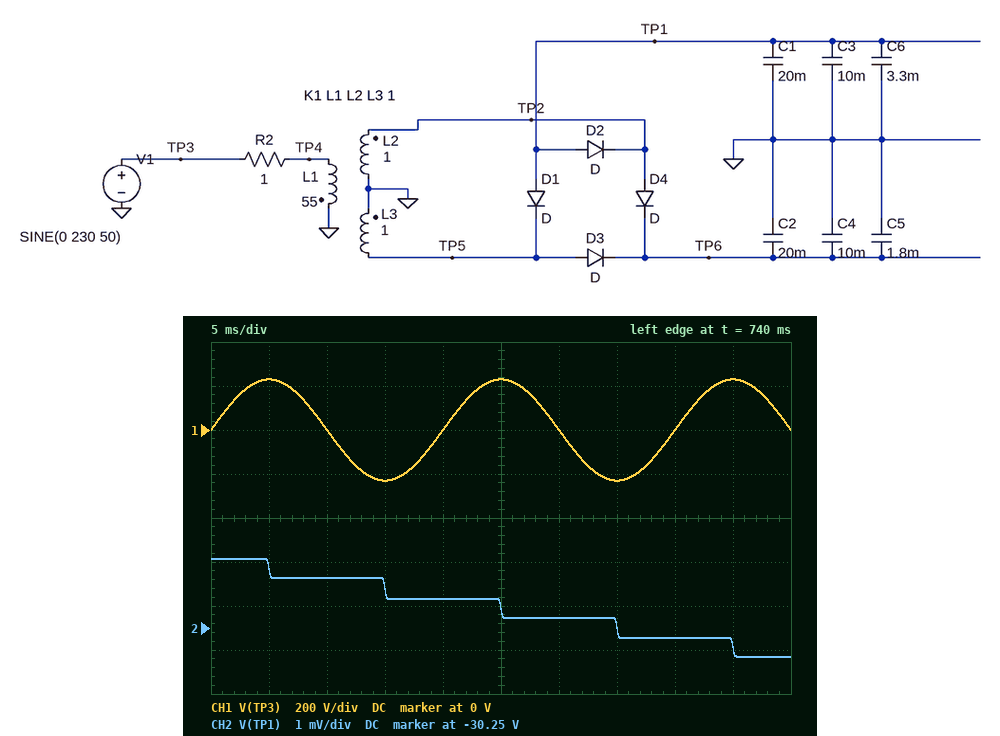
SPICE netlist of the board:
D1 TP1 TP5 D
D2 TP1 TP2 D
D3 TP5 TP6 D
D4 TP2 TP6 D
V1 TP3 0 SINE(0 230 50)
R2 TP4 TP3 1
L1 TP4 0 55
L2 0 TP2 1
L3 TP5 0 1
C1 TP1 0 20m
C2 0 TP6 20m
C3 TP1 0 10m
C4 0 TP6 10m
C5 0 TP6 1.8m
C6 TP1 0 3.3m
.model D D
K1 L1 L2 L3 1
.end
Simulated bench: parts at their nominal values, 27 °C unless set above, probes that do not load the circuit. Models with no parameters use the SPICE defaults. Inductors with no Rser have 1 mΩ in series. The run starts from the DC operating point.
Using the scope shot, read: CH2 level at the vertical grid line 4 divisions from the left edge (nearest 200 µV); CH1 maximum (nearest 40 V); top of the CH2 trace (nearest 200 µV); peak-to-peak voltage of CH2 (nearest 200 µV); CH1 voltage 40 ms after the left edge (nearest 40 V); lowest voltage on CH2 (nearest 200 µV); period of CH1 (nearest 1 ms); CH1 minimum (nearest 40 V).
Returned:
-30.2484 V
240 V
-30.2474 V
2.2 mV
0 V
-30.2496 V
20 ms
-240 V
